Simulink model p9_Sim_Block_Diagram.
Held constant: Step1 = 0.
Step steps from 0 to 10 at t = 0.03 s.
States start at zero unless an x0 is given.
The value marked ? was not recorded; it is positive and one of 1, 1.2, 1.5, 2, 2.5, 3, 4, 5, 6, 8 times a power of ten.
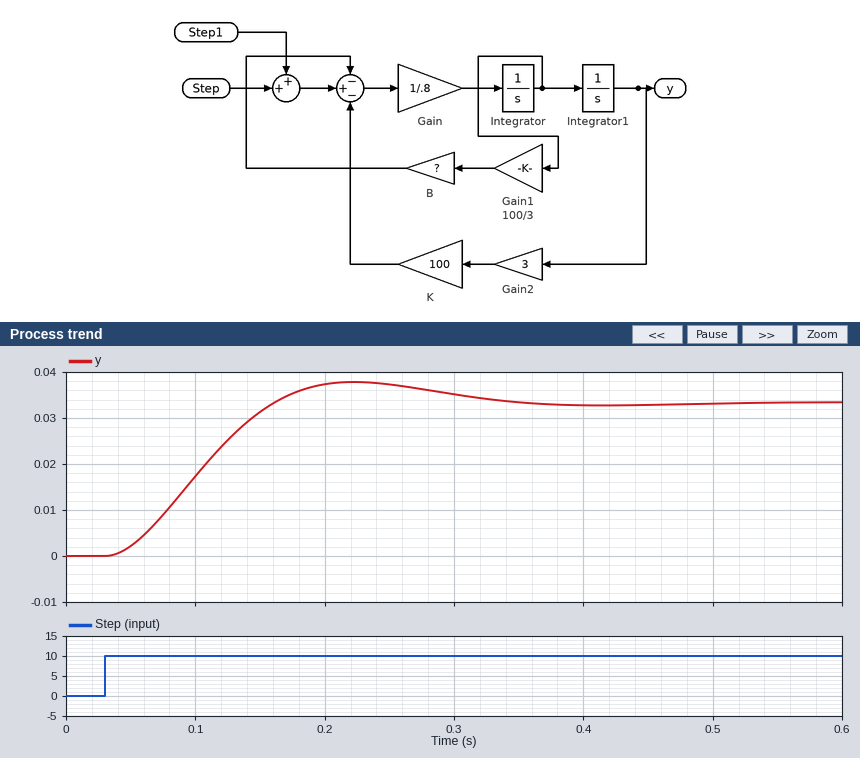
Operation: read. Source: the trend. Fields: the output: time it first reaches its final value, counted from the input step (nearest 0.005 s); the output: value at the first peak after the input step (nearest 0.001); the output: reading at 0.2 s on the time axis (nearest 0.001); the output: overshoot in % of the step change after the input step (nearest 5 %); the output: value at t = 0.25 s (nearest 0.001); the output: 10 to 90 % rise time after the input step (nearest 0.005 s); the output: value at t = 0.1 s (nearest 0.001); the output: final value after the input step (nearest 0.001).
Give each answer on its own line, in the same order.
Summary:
0.130 s
0.038
0.037
15 %
0.037
0.090 s
0.017
0.033
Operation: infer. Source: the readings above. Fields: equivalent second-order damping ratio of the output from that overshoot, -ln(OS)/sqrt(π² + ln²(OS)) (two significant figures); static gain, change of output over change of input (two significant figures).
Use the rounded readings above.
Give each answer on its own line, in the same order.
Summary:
0.52
0.0033
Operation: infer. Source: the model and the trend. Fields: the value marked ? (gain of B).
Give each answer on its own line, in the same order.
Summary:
0.5
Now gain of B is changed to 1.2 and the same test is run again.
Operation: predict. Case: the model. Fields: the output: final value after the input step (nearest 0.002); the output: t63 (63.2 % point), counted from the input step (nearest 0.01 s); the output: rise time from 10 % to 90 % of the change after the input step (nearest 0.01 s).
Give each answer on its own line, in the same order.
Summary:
0.034
0.14 s
0.25 s
